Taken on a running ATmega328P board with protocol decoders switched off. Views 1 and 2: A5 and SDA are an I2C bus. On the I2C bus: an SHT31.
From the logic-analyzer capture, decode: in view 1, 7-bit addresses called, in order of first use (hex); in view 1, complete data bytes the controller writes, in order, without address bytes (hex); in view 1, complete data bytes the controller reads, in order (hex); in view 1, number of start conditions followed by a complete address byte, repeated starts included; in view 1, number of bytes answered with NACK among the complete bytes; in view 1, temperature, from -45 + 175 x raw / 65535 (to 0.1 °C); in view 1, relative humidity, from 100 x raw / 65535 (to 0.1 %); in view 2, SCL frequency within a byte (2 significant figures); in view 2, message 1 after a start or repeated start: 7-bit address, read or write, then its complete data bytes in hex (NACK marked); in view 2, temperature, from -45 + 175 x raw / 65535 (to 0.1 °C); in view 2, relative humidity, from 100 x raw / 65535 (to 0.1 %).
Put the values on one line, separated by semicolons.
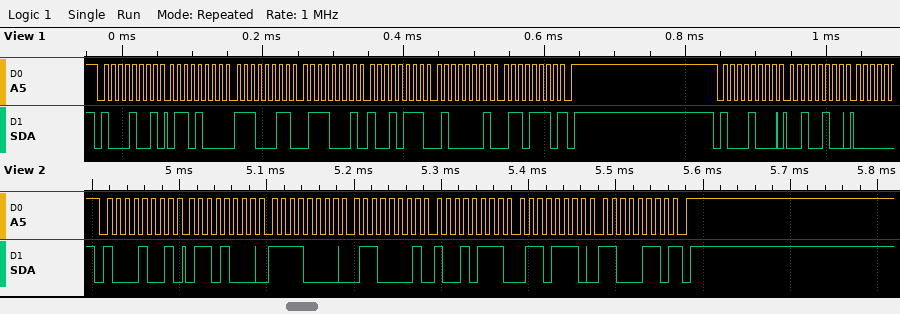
0x44; 24; 68 E3 71 97 41 6E; 2; 1; 26.7 °C; 59.1 %; 100 kHz; 0x44 read: 68 F0 61 97 6E C6 NACK; 26.7 °C; 59.2 %
